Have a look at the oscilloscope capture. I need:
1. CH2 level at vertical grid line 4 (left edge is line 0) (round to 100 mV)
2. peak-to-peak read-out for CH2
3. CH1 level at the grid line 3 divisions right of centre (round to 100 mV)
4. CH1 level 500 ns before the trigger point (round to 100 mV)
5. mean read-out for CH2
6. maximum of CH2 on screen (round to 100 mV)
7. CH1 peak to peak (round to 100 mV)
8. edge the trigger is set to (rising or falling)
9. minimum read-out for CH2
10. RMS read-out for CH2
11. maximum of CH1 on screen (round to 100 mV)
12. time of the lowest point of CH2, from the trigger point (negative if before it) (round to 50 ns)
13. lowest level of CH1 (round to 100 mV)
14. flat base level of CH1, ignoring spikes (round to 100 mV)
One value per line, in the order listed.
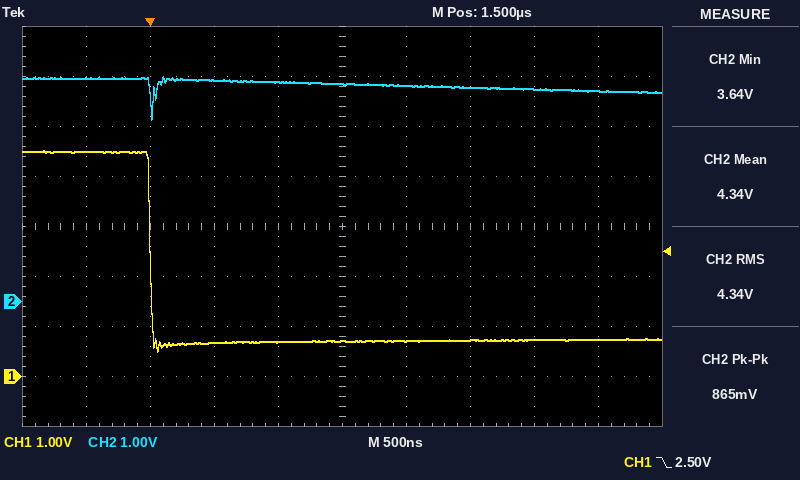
4.4 V
865 mV
700 mV
4.5 V
4.34 V
4.5 V
4.0 V
falling
3.64 V
4.34 V
4.5 V
0 ns
500 mV
700 mV
